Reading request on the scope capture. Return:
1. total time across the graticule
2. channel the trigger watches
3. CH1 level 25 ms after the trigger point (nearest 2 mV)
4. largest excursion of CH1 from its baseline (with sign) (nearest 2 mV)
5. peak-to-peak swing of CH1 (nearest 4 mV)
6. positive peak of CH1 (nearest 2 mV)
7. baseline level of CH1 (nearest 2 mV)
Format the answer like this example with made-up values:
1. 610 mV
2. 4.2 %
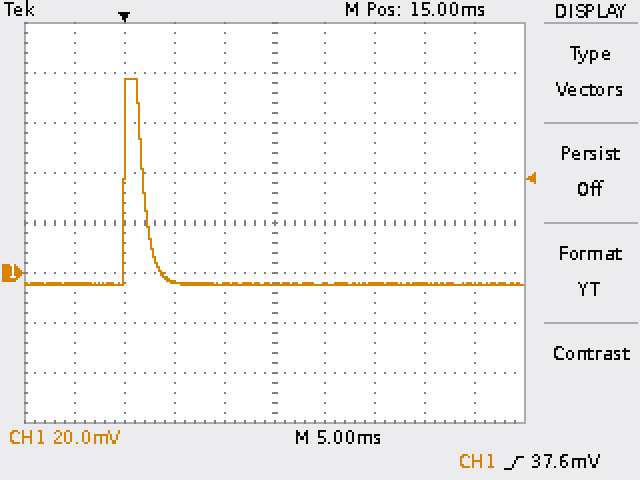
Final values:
1. 50 ms
2. CH1
3. -4 mV
4. +82 mV
5. 84 mV
6. 78 mV
7. -4 mV
